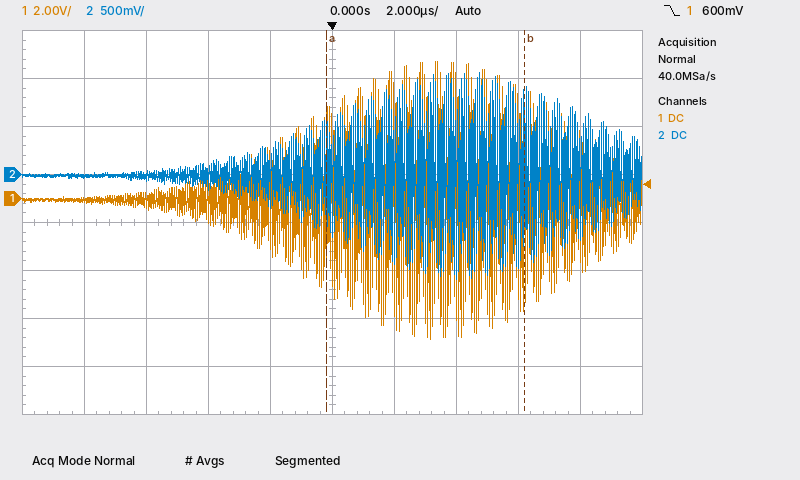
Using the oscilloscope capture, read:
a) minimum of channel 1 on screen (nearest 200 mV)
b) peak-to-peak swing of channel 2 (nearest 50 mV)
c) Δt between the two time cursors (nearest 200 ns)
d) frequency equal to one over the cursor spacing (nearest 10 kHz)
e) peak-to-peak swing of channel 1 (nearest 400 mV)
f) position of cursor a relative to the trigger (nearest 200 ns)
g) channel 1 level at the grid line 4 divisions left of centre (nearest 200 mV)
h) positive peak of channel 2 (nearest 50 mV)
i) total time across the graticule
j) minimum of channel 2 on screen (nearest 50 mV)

-5.8 V
2.15 V
6.4 µs
160 kHz
11.6 V
-200 ns
0.0 V
1.05 V
20 µs
-1.10 V
